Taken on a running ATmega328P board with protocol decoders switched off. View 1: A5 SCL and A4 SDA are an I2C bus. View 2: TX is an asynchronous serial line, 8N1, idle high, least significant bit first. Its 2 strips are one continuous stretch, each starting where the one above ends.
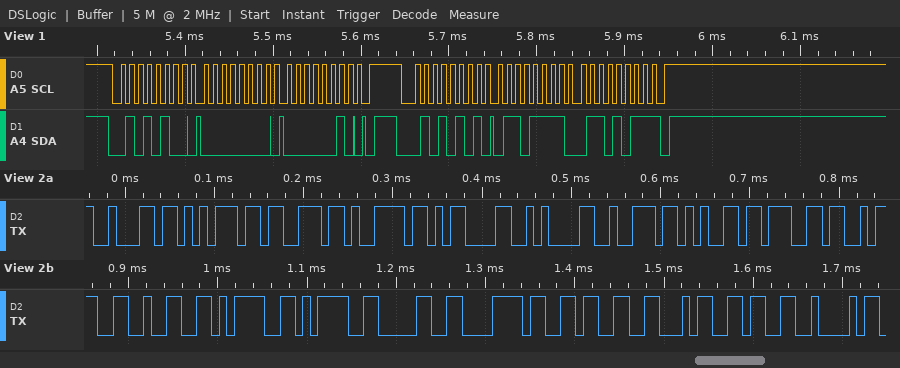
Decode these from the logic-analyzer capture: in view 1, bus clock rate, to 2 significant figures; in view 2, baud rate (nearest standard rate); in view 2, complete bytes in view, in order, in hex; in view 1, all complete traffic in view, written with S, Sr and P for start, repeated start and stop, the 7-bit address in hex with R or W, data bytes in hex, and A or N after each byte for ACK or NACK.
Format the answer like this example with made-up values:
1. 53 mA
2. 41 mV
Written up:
1. 100 kHz
2. 115200 baud
3. 0x62 0x75 0x73 0x79 0x0D 0x0A 0x72 0x65 0x67 0x3A 0x32 0x3D 0x3D 0x30 0x78 0x36 0x46 0x36 0x42
4. S 2AW A 00 A 02 A P S 2AR A 6F A 6B N P
